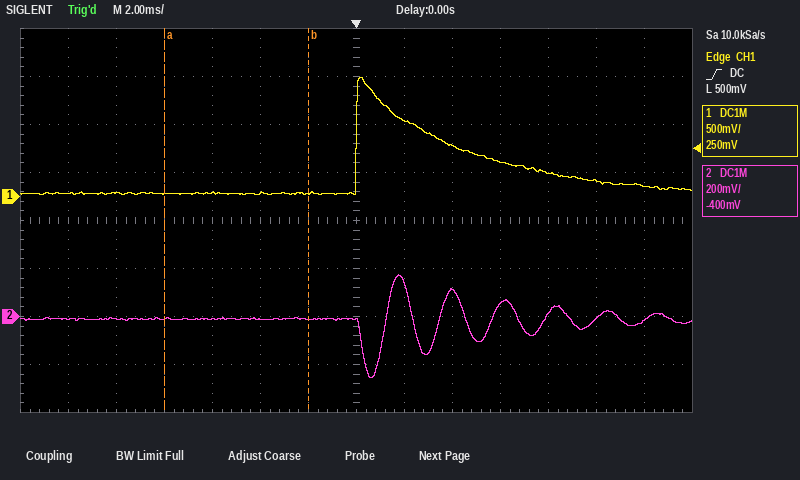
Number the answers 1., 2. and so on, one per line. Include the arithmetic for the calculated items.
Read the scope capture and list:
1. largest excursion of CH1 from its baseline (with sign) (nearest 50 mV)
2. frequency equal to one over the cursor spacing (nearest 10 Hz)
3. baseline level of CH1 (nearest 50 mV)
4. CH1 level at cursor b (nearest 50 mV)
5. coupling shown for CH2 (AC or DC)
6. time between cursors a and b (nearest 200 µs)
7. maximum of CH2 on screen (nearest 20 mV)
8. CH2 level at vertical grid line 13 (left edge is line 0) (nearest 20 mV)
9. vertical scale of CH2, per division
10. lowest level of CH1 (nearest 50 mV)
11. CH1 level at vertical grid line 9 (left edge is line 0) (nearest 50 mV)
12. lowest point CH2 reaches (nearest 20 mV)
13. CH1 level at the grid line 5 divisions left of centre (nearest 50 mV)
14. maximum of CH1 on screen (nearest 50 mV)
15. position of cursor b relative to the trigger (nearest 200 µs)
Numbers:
1. 1.25 V − (50 mV) = +1.20 V
2. 1 / 6.0 ms ≈ 170 Hz
3. 50 mV
4. 50 mV
5. DC
6. 6.0 ms
7. 180 mV
8. -20 mV
9. 200 mV
10. 0 mV
11. 550 mV
12. -260 mV
13. 50 mV
14. 1.25 V
15. -2.0 ms
